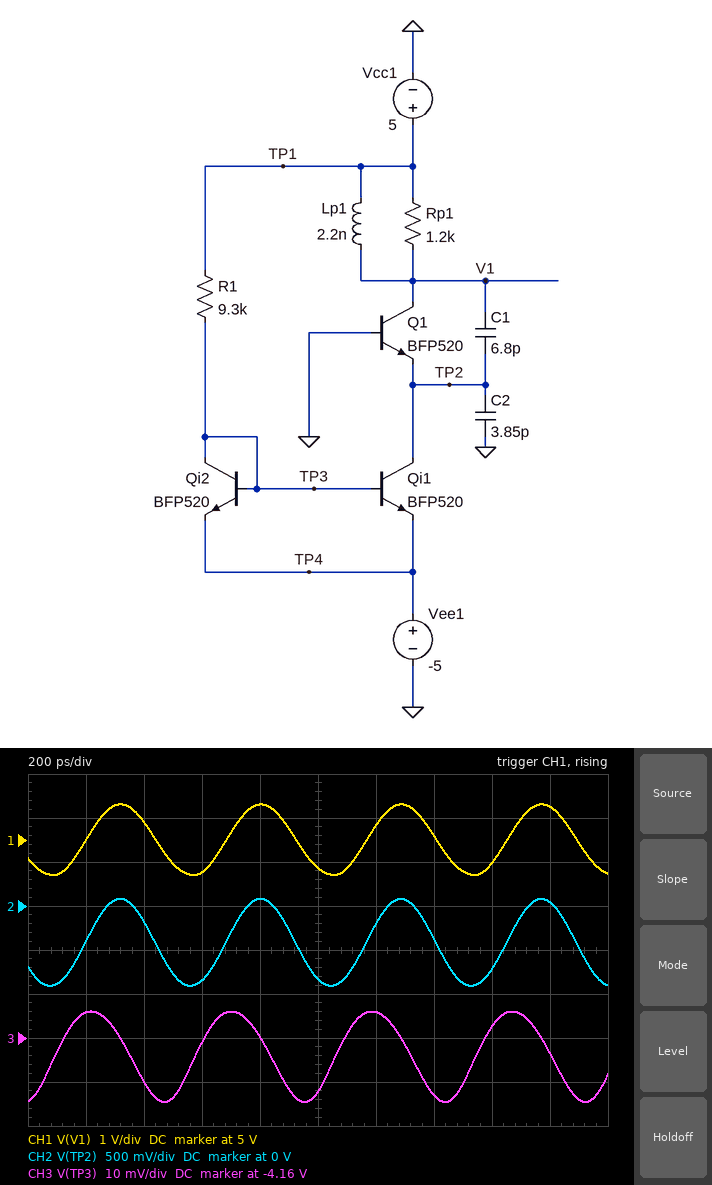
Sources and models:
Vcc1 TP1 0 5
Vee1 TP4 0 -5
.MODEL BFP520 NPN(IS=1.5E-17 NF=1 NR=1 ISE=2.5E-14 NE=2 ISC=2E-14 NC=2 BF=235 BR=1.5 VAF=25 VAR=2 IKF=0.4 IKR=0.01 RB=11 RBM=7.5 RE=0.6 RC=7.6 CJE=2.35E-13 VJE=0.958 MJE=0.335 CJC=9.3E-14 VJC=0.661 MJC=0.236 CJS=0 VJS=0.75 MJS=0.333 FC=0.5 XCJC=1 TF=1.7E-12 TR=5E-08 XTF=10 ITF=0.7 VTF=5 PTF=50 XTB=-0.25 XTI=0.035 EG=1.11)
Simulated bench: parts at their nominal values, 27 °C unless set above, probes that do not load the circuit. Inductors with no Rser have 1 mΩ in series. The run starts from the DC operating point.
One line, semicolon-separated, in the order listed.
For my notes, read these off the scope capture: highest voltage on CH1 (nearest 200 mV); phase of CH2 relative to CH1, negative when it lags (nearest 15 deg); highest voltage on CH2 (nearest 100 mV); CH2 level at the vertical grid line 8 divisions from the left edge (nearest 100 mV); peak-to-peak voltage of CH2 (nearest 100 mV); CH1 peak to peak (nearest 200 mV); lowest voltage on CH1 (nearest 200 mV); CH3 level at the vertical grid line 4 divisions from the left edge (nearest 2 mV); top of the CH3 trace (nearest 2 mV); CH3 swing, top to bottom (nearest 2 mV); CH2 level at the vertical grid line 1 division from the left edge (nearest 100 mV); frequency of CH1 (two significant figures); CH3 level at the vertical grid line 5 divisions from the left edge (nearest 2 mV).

5.8 V; 0 deg; 100 mV; -700 mV; 1.0 V; 1.6 V; 4.2 V; -4.160 V; -4.154 V; 20 mV; -400 mV; 2.1 GHz; -4.172 V
